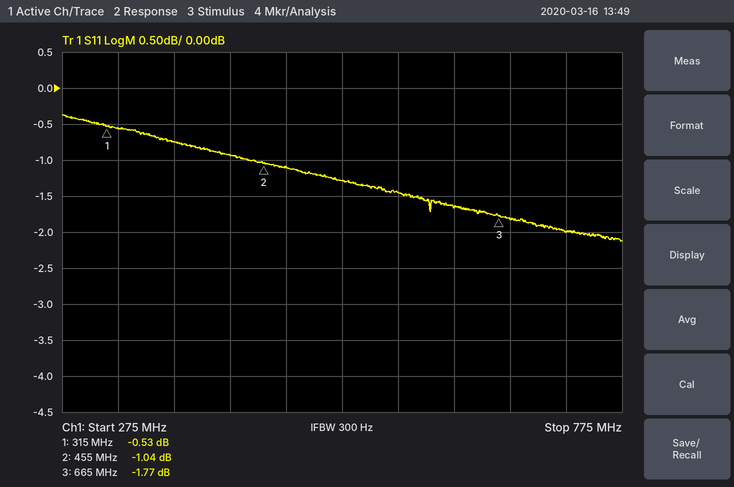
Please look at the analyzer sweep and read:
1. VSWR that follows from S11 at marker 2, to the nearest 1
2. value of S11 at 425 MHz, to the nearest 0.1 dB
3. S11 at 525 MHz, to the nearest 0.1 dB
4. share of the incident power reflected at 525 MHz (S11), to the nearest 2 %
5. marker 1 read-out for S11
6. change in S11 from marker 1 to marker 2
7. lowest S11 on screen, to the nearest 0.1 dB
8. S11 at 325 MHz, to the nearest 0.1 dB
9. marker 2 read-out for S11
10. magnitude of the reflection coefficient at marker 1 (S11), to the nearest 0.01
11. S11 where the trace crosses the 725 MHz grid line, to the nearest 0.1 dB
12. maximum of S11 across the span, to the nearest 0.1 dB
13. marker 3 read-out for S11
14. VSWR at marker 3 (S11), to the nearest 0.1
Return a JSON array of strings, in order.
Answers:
["17", "-0.9 dB", "-1.3 dB", "74 %", "-0.53 dB", "-0.51 dB", "-2.1 dB", "-0.6 dB", "-1.04 dB", "0.94", "-2.0 dB", "-0.4 dB", "-1.77 dB", "9.8"]
